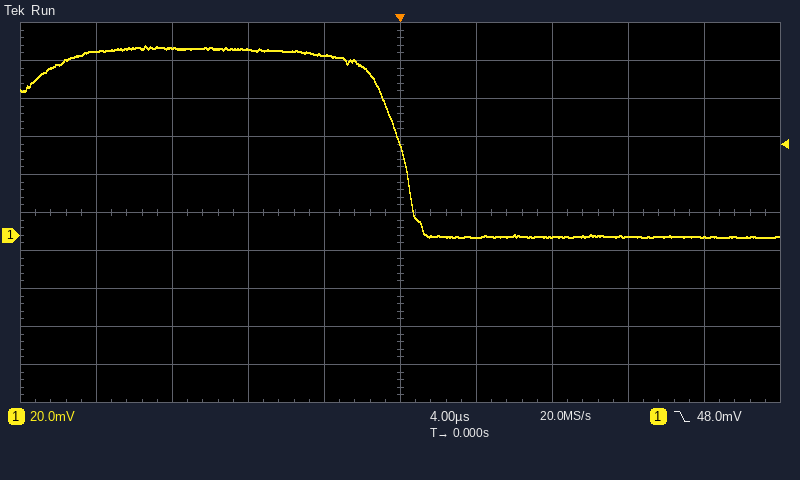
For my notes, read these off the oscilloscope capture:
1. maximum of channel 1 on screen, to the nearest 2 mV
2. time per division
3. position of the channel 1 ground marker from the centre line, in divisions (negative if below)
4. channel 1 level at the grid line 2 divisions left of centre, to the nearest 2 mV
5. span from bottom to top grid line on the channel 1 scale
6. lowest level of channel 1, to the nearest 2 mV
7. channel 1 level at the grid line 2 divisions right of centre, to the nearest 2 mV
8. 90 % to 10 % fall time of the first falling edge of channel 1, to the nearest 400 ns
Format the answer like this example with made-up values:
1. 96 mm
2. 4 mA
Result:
1. 100 mV
2. 4 µs
3. -0.6 div
4. 98 mV
5. 200 mV
6. -2 mV
7. 0 mV
8. 2.8 µs
